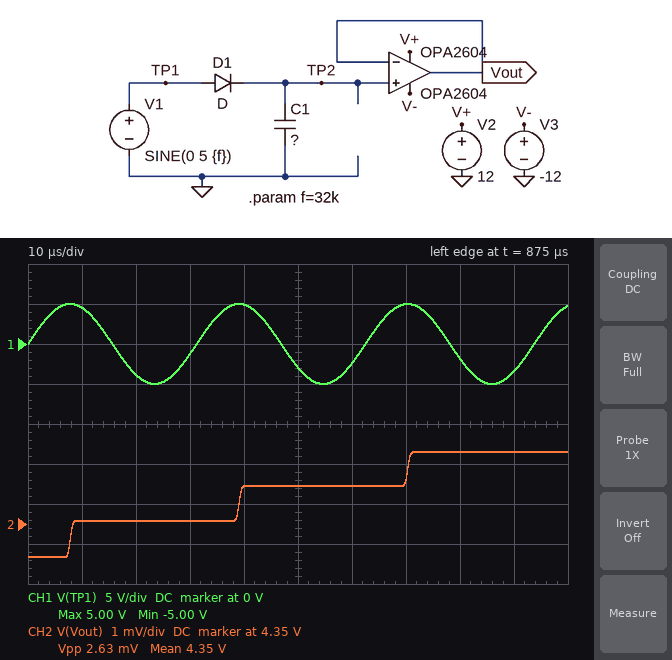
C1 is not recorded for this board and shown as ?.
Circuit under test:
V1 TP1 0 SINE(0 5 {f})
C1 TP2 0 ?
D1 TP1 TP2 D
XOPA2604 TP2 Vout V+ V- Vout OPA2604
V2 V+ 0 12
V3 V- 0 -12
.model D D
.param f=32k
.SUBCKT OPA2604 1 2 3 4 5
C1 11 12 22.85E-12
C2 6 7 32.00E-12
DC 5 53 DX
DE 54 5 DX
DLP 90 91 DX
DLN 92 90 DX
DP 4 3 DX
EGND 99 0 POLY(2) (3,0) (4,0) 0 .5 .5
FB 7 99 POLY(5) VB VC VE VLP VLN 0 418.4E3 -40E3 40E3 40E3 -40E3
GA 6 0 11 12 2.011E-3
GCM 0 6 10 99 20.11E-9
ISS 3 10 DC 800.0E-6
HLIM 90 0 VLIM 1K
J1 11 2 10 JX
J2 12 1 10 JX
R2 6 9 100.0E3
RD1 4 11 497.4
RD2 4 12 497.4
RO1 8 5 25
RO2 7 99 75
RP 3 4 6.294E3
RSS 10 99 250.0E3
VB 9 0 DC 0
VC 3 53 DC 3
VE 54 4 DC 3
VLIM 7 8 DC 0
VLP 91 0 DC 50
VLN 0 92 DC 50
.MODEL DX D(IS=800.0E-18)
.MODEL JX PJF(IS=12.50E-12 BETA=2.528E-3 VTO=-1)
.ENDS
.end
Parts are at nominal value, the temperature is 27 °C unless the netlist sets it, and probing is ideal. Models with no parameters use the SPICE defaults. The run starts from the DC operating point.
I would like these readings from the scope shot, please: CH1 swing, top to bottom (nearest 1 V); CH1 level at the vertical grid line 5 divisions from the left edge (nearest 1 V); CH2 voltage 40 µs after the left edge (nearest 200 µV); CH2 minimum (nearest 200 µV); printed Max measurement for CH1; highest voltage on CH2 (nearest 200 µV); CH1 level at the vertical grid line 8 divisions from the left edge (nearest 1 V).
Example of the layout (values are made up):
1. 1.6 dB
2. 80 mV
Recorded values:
1. 10 V
2. -3 V
3. 4.3510 V
4. 4.3492 V
5. 5.00 V
6. 4.3518 V
7. -2 V
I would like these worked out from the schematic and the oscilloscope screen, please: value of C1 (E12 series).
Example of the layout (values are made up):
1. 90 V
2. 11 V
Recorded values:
1. 820 nF
